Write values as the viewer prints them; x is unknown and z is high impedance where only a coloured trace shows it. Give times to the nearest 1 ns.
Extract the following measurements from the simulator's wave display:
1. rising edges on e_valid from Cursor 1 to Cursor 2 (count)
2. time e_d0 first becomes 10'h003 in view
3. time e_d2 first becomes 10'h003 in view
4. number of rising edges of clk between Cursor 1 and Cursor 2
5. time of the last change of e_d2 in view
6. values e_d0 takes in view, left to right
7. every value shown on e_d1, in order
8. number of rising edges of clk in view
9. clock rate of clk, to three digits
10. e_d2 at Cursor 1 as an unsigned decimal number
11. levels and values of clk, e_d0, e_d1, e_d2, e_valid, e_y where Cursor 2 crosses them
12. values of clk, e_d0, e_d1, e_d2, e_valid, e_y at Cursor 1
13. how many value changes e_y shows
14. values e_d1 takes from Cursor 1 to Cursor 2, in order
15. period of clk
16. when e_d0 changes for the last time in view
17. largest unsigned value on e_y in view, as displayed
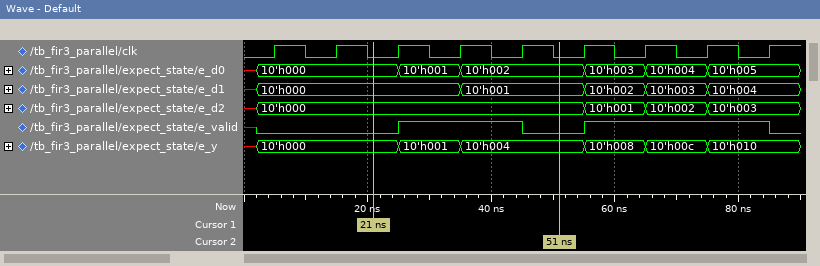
1
55 ns
75 ns
3
75 ns
x, 10'h000, 10'h001, 10'h002, 10'h003, 10'h004, 10'h005
x, 10'h000, 10'h001, 10'h002, 10'h003, 10'h004
9
100 MHz
0
clk=0, e_d0=10'h002, e_d1=10'h001, e_d2=10'h000, e_valid=0, e_y=10'h004
clk=0, e_d0=10'h000, e_d1=10'h000, e_d2=10'h000, e_valid=0, e_y=10'h000
6
10'h000, 10'h001
10 ns
75 ns
10'h010
